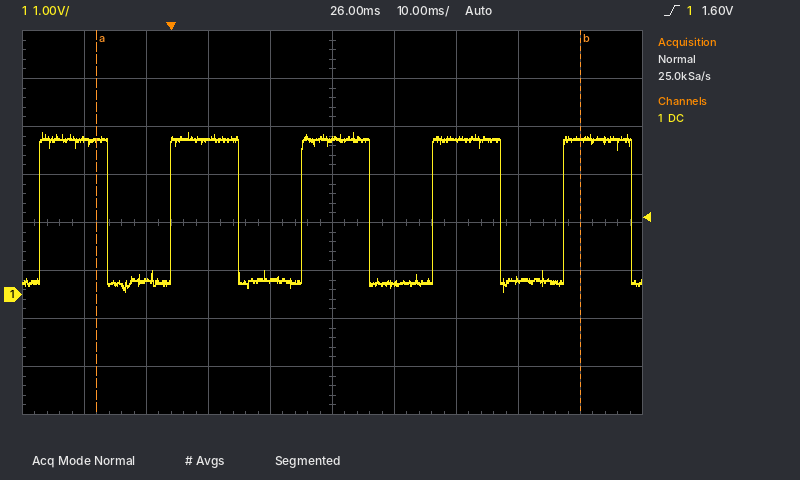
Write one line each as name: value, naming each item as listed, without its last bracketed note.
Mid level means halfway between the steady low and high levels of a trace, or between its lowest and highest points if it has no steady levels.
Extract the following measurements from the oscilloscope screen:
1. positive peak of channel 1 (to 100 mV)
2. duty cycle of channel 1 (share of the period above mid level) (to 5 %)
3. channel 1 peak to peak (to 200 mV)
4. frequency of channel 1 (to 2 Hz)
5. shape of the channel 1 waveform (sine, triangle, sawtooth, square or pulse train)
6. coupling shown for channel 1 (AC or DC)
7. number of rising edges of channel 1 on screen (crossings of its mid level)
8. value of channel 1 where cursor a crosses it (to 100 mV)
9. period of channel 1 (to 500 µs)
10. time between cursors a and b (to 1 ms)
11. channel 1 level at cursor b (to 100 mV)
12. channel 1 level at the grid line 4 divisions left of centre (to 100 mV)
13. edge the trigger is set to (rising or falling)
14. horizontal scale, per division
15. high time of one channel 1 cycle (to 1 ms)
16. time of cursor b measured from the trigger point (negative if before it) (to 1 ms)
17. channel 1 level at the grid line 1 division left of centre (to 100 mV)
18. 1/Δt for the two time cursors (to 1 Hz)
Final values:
positive peak of channel 1: 3.4 V
duty cycle of channel 1 (share of the period above mid level): 50 %
channel 1 peak to peak: 3.4 V
frequency of channel 1: 48 Hz
shape of the channel 1 waveform: square
coupling shown for channel 1: DC
number of rising edges of channel 1 on screen: 5
value of channel 1 where cursor a crosses it: 3.2 V
period of channel 1: 21.0 ms
time between cursors a and b: 78 ms
channel 1 level at cursor b: 3.2 V
channel 1 level at the grid line 4 divisions left of centre: 3.2 V
edge the trigger is set to: rising
horizontal scale, per division: 10 ms
high time of one channel 1 cycle: 11 ms
time of cursor b measured from the trigger point (negative if before it): +66 ms
channel 1 level at the grid line 1 division left of centre: 300 mV
1/Δt for the two time cursors: 13 Hz
